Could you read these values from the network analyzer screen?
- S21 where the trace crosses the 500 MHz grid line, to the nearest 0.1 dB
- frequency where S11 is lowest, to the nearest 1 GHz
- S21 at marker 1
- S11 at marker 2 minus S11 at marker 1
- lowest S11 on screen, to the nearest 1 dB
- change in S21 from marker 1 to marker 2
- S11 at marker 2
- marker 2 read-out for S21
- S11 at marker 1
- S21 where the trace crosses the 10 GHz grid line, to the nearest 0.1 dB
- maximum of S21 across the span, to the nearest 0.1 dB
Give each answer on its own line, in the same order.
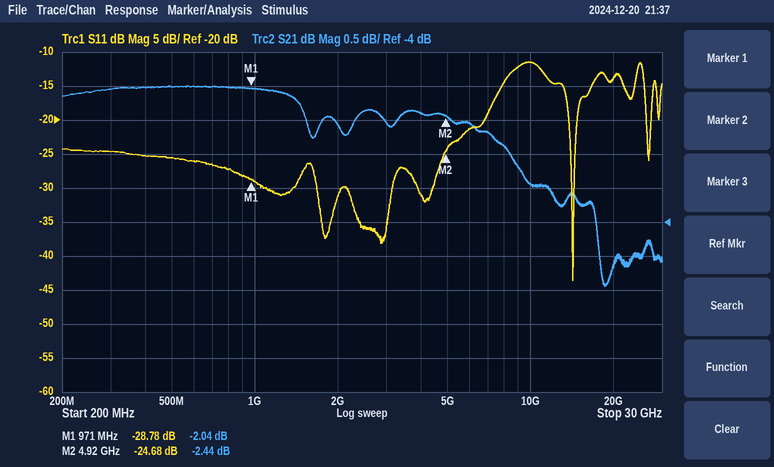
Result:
-2.0 dB
14 GHz
-2.04 dB
4.10 dB
-44 dB
-0.40 dB
-24.68 dB
-2.44 dB
-28.78 dB
-3.4 dB
-2.0 dB
